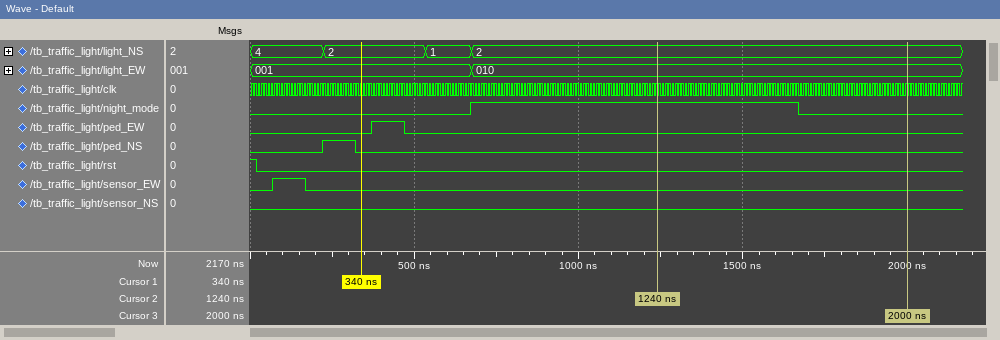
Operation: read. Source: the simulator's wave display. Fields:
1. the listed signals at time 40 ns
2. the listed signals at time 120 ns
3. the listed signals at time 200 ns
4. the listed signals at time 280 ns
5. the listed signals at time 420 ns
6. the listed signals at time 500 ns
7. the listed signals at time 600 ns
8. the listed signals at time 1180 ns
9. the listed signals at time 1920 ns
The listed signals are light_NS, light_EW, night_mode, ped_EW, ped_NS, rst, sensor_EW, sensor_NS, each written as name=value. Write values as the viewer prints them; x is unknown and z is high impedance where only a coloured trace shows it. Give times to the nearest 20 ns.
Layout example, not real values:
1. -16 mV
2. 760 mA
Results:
1. light_NS=4, light_EW=001, night_mode=0, ped_EW=0, ped_NS=0, rst=0, sensor_EW=0, sensor_NS=0
2. light_NS=4, light_EW=001, night_mode=0, ped_EW=0, ped_NS=0, rst=0, sensor_EW=1, sensor_NS=0
3. light_NS=4, light_EW=001, night_mode=0, ped_EW=0, ped_NS=0, rst=0, sensor_EW=0, sensor_NS=0
4. light_NS=2, light_EW=001, night_mode=0, ped_EW=0, ped_NS=1, rst=0, sensor_EW=0, sensor_NS=0
5. light_NS=2, light_EW=001, night_mode=0, ped_EW=1, ped_NS=0, rst=0, sensor_EW=0, sensor_NS=0
6. light_NS=2, light_EW=001, night_mode=0, ped_EW=0, ped_NS=0, rst=0, sensor_EW=0, sensor_NS=0
7. light_NS=1, light_EW=001, night_mode=0, ped_EW=0, ped_NS=0, rst=0, sensor_EW=0, sensor_NS=0
8. light_NS=2, light_EW=010, night_mode=1, ped_EW=0, ped_NS=0, rst=0, sensor_EW=0, sensor_NS=0
9. light_NS=2, light_EW=010, night_mode=0, ped_EW=0, ped_NS=0, rst=0, sensor_EW=0, sensor_NS=0
